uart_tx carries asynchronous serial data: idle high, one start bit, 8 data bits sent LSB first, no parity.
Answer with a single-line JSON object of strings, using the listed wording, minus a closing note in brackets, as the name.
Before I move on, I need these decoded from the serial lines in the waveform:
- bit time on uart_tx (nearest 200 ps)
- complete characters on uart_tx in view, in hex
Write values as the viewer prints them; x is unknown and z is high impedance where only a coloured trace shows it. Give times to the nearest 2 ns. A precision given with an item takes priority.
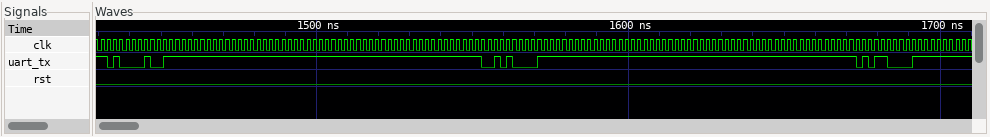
{"bit time on uart_tx": "2000 ps", "complete characters on uart_tx in view, in hex": "21, 0A, 0D"}
